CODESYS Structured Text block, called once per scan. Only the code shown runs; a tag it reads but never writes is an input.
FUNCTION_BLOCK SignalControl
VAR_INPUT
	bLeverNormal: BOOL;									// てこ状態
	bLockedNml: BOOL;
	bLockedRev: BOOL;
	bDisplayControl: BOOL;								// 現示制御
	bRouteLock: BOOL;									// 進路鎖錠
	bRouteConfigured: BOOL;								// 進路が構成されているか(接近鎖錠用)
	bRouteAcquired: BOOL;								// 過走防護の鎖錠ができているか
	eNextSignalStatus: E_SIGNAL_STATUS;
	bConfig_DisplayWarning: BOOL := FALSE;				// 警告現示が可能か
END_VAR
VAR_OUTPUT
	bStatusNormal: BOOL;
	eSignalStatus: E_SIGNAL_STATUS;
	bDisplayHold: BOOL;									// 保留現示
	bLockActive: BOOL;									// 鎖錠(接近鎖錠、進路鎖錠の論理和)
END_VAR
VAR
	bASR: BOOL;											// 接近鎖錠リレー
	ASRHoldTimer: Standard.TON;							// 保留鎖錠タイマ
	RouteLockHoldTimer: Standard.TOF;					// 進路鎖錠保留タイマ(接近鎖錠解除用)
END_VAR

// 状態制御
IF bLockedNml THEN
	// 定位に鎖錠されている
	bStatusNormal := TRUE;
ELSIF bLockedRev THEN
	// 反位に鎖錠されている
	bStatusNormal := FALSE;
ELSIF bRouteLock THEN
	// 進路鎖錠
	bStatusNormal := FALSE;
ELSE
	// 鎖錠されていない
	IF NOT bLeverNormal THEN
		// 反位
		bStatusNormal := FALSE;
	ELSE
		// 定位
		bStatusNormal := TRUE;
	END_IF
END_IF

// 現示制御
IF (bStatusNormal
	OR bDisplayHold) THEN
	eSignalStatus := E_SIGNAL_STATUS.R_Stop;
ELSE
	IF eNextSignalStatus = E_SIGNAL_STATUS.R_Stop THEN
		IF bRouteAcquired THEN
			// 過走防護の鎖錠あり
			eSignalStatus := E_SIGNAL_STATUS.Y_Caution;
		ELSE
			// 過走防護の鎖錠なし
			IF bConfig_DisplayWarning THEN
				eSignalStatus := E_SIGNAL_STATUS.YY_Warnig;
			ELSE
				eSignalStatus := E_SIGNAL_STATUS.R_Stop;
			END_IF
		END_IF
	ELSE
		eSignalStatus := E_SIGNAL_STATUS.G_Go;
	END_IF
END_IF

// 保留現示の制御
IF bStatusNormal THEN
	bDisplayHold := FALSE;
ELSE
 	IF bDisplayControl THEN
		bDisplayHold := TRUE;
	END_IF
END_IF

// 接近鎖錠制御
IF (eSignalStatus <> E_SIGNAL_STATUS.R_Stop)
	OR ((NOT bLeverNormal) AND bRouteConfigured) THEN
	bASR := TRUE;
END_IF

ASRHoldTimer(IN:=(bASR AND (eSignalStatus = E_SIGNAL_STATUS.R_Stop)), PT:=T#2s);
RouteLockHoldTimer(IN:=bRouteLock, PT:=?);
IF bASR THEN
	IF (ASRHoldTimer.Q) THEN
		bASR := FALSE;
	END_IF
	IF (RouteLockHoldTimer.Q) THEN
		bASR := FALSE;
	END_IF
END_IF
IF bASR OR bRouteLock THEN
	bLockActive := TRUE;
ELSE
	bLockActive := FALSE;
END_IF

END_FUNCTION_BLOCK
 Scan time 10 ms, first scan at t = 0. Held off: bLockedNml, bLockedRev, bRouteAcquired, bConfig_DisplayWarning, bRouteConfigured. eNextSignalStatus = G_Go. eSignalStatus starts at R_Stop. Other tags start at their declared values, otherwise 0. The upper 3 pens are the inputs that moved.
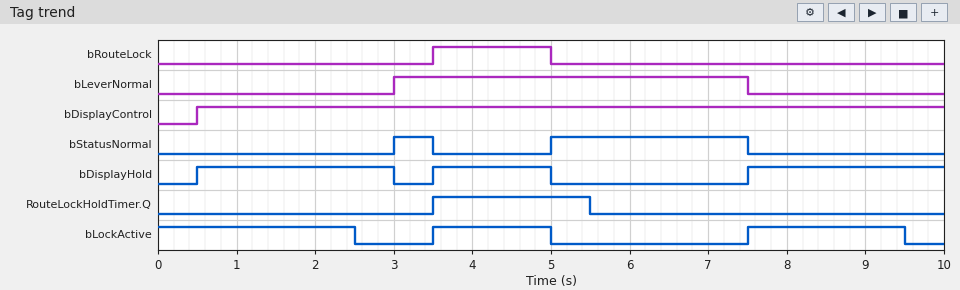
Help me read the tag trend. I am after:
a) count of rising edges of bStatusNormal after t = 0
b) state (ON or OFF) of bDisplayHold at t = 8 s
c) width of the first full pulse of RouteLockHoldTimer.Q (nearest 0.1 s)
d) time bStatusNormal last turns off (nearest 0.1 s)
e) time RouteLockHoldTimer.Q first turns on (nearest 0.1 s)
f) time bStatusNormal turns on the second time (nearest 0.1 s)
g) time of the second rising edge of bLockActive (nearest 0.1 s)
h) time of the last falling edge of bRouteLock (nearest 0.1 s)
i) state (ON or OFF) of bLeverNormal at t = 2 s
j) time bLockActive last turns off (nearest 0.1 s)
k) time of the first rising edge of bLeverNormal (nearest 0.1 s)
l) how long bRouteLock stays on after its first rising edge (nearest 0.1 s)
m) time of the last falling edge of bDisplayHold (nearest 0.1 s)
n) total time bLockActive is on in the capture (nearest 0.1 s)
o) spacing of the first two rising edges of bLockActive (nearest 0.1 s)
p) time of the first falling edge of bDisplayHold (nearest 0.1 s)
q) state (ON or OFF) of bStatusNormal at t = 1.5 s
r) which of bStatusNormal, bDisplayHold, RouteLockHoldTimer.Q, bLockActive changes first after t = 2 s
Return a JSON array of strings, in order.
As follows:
["2", "ON", "2.0 s", "7.5 s", "3.5 s", "5.0 s", "7.5 s", "5.0 s", "OFF", "9.5 s", "3.0 s", "1.5 s", "5.0 s", "6.0 s", "4.0 s", "3.0 s", "OFF", "bLockActive"]
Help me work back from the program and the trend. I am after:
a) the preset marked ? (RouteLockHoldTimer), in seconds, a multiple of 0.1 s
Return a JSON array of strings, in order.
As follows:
["0.5 s"]
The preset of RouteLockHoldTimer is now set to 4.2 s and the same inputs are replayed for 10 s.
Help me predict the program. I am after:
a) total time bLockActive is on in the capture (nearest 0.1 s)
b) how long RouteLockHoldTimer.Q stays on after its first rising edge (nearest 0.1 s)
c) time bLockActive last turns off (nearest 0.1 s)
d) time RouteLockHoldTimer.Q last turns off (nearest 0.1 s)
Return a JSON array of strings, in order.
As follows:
["4.0 s", "5.7 s", "5.0 s", "9.2 s"]
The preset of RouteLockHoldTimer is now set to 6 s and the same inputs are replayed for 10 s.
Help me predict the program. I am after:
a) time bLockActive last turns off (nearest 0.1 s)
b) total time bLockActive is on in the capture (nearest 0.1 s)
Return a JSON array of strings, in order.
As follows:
["5.0 s", "4.0 s"]
